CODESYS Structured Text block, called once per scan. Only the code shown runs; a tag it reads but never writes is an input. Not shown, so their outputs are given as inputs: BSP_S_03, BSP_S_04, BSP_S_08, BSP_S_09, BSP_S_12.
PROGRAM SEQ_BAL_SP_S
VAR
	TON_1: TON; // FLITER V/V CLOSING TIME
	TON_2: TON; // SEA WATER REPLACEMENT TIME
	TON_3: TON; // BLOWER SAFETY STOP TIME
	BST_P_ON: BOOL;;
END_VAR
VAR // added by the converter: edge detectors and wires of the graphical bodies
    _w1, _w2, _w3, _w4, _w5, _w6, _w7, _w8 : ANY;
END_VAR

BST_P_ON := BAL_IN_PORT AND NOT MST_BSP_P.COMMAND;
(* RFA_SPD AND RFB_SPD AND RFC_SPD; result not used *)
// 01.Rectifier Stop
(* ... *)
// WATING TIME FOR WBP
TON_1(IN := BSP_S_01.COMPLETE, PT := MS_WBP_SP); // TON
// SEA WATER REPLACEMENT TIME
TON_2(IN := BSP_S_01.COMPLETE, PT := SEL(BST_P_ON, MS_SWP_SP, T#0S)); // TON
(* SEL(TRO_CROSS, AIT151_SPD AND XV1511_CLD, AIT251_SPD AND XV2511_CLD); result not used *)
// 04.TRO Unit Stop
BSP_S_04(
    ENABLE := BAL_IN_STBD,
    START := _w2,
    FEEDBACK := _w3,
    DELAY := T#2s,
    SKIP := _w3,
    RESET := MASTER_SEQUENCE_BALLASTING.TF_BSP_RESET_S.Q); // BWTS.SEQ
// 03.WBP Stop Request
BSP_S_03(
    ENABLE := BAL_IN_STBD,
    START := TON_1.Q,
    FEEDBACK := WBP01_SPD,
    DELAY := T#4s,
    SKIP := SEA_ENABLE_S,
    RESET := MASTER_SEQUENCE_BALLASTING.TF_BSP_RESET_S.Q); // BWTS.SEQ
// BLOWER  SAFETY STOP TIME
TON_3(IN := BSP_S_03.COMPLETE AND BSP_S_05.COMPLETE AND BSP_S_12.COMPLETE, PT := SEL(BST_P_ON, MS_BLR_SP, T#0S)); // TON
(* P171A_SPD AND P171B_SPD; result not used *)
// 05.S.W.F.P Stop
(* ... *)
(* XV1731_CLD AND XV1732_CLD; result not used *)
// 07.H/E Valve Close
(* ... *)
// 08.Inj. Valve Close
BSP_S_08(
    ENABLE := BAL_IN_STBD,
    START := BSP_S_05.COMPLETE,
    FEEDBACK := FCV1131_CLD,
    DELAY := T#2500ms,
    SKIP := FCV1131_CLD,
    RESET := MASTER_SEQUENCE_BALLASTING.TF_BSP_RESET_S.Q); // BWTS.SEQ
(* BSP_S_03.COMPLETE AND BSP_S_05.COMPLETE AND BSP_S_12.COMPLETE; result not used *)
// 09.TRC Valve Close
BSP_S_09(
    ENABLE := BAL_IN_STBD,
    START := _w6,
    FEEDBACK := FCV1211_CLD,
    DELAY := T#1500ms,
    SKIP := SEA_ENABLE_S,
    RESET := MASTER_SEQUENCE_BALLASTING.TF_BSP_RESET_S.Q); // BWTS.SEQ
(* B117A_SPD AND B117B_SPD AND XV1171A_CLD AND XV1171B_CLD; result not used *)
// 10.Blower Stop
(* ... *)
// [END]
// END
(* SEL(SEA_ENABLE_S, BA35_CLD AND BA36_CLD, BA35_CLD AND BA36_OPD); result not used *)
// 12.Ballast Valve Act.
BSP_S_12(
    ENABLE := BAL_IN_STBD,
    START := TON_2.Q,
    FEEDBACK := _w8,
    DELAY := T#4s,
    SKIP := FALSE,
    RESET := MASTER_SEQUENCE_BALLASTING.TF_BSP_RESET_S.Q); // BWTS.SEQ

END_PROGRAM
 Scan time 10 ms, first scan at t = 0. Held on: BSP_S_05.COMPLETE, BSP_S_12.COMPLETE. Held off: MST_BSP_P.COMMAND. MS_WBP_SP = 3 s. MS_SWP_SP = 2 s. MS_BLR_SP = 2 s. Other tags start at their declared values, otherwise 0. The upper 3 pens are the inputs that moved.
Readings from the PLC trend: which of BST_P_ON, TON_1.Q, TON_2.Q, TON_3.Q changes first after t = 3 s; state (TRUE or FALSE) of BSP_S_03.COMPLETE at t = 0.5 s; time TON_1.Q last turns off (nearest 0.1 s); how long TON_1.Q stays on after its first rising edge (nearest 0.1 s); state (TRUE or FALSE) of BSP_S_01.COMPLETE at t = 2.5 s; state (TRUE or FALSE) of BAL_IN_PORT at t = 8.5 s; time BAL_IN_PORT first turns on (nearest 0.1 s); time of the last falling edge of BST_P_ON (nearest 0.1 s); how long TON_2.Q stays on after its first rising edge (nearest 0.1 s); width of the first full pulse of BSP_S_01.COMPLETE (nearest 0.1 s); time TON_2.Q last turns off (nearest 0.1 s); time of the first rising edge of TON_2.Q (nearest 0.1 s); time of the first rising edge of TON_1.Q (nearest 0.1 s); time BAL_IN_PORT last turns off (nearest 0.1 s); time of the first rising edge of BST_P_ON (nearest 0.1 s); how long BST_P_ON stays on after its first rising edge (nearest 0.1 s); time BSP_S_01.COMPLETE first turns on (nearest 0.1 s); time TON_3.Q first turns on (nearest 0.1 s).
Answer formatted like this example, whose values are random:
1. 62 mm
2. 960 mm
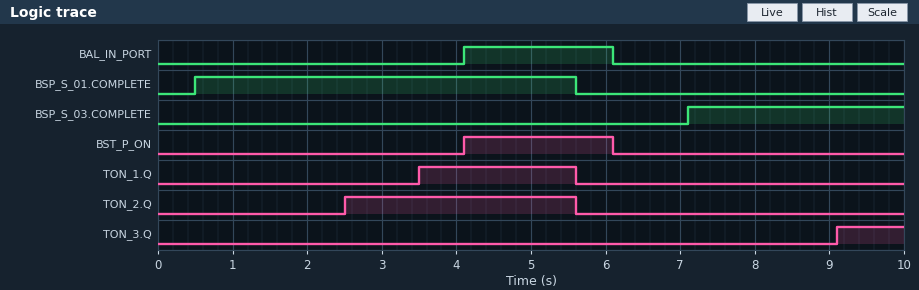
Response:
1. TON_1.Q
2. FALSE
3. 5.6 s
4. 2.1 s
5. TRUE
6. FALSE
7. 4.1 s
8. 6.1 s
9. 3.1 s
10. 5.1 s
11. 5.6 s
12. 2.5 s
13. 3.5 s
14. 6.1 s
15. 4.1 s
16. 2.0 s
17. 0.5 s
18. 9.1 s
